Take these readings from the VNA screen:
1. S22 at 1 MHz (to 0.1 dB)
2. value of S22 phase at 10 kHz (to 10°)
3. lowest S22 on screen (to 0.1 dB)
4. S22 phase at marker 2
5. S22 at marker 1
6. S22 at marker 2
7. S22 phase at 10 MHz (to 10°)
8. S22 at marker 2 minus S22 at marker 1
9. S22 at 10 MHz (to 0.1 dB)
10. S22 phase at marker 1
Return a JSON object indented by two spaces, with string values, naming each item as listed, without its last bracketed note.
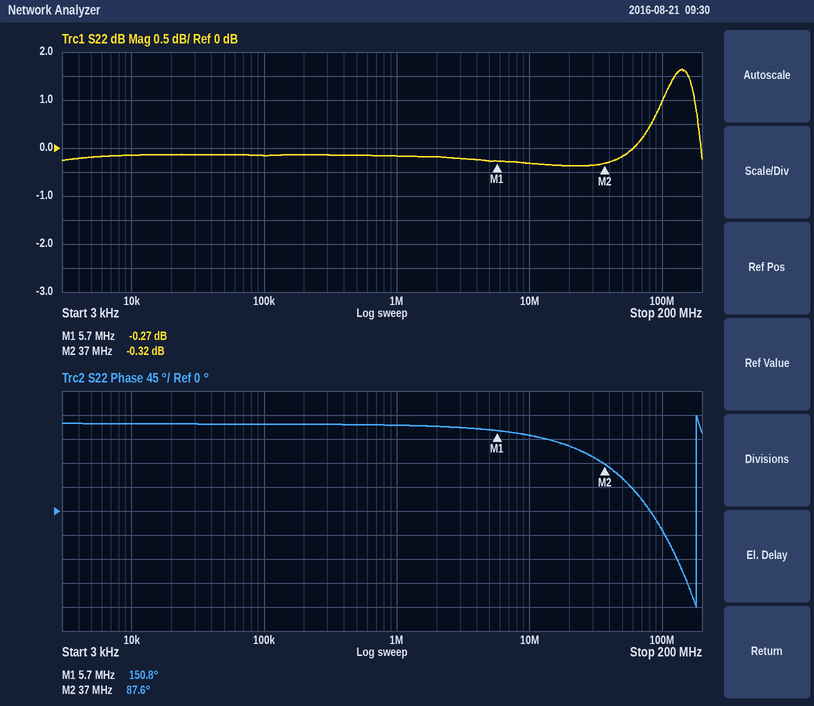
{
  "S22 at 1 MHz": "-0.2 dB",
  "value of S22 phase at 10 kHz": "160°",
  "lowest S22 on screen": "-0.4 dB",
  "S22 phase at marker 2": "87.6°",
  "S22 at marker 1": "-0.27 dB",
  "S22 at marker 2": "-0.32 dB",
  "S22 phase at 10 MHz": "140°",
  "S22 at marker 2 minus S22 at marker 1": "-0.05 dB",
  "S22 at 10 MHz": "-0.3 dB",
  "S22 phase at marker 1": "150.8°"
}
